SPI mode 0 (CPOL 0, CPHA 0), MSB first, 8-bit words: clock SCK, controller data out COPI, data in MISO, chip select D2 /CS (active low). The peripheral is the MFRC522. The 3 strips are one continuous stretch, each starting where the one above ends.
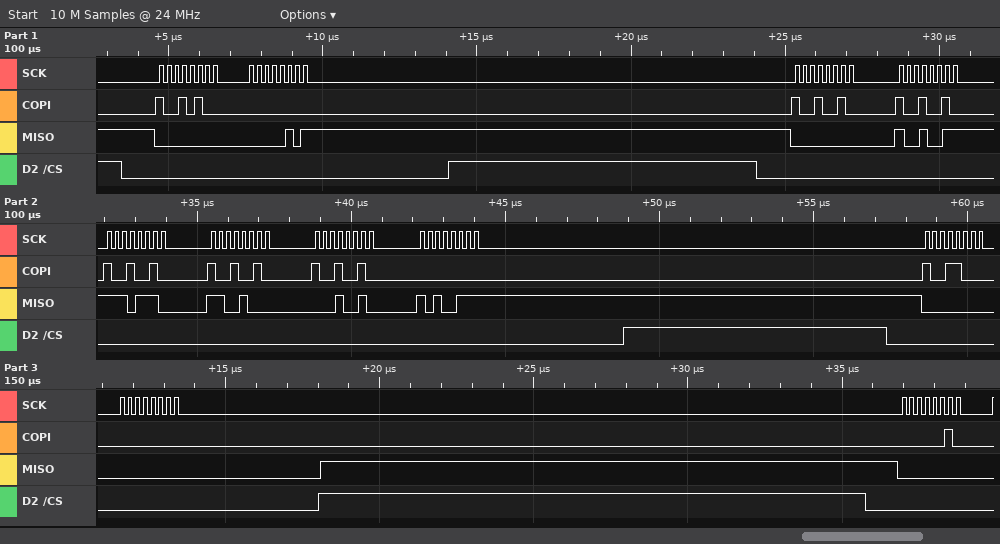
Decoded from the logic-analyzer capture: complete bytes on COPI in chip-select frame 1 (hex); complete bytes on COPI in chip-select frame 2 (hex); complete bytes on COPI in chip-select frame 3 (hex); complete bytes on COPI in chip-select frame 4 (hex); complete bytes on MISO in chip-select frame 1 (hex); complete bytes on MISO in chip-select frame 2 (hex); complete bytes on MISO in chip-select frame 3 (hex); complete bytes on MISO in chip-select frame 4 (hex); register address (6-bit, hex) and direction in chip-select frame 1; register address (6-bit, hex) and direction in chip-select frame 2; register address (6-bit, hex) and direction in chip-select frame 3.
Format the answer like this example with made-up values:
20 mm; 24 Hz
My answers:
94 00; 92 92 92 92 92 00; 98 00; 02; 00 05; 00 93 EE C8 12 A7; 00 00; 00; 0x0A read; 0x09 read; 0x0C read
